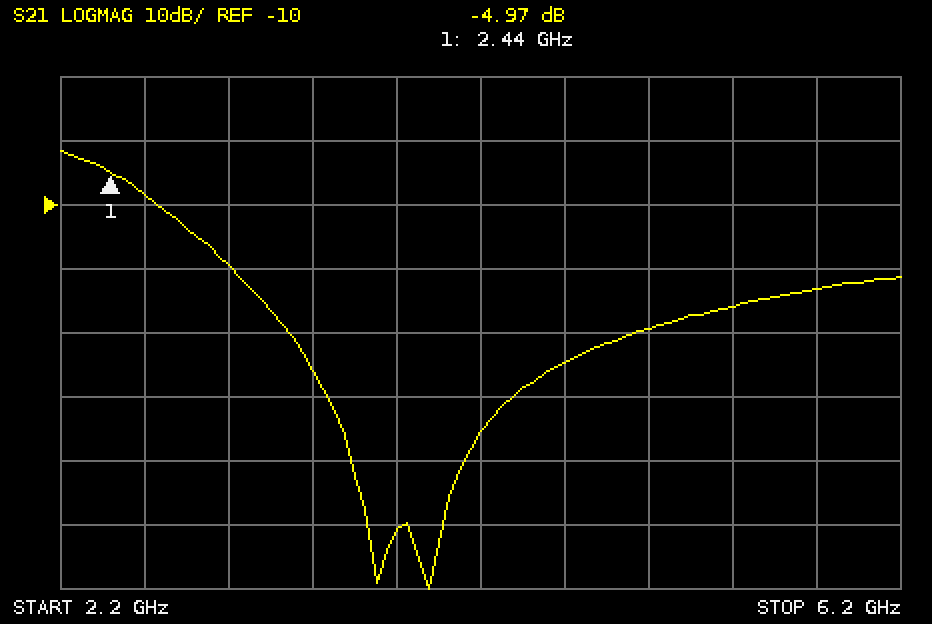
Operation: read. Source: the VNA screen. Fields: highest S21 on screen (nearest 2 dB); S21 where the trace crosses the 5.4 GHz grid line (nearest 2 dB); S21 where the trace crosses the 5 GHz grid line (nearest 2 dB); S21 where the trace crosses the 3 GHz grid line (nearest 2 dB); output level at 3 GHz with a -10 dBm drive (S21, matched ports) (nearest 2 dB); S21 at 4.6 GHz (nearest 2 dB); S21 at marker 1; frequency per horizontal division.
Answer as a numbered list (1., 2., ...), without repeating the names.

1. -2 dB
2. -26 dB
3. -30 dB
4. -20 dB
5. -30 dBm
6. -34 dB
7. -4.97 dB
8. 400 MHz
